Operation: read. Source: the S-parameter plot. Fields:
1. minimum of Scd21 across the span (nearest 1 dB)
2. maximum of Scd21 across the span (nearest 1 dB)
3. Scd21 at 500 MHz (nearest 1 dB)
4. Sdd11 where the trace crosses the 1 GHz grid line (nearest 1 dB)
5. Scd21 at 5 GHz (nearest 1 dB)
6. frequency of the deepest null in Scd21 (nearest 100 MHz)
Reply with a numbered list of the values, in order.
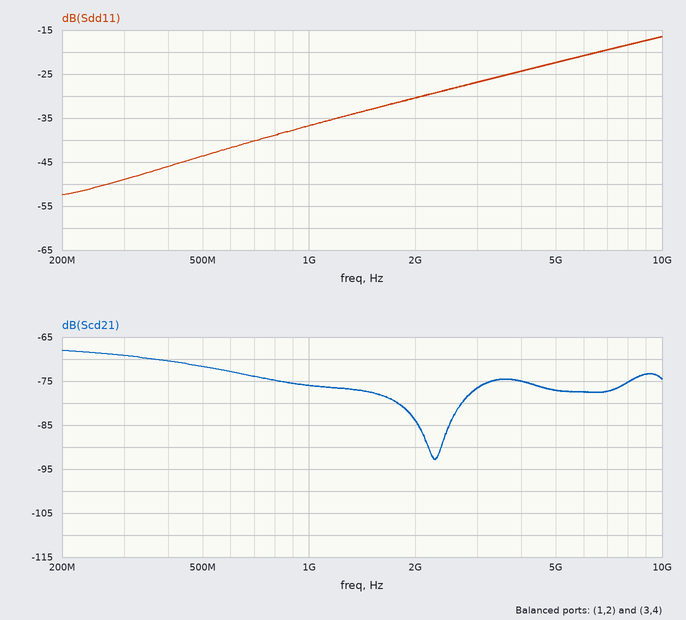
1. -93 dB
2. -68 dB
3. -72 dB
4. -37 dB
5. -77 dB
6. 2.3 GHz
